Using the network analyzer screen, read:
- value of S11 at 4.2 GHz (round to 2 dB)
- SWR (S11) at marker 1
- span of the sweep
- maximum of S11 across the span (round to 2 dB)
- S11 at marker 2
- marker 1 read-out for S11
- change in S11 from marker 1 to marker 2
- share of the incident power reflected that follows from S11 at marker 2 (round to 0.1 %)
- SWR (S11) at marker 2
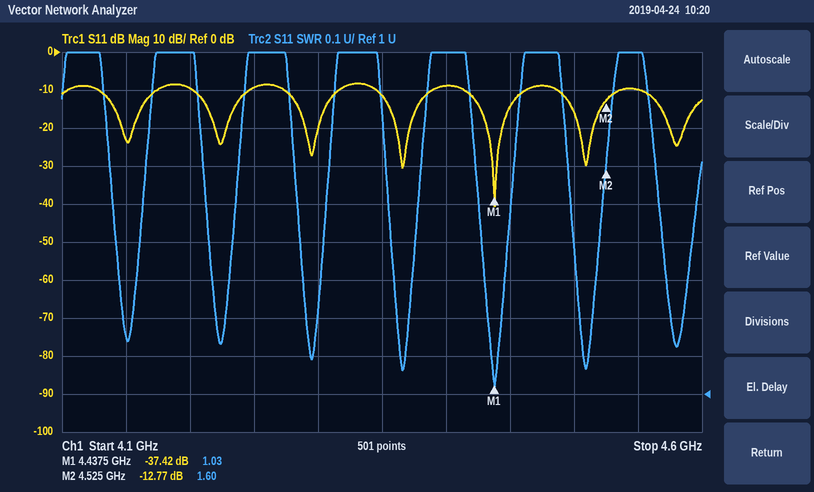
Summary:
-10 dB
1.03
500 MHz
-8 dB
-12.77 dB
-37.42 dB
24.65 dB
5.3 %
1.60
